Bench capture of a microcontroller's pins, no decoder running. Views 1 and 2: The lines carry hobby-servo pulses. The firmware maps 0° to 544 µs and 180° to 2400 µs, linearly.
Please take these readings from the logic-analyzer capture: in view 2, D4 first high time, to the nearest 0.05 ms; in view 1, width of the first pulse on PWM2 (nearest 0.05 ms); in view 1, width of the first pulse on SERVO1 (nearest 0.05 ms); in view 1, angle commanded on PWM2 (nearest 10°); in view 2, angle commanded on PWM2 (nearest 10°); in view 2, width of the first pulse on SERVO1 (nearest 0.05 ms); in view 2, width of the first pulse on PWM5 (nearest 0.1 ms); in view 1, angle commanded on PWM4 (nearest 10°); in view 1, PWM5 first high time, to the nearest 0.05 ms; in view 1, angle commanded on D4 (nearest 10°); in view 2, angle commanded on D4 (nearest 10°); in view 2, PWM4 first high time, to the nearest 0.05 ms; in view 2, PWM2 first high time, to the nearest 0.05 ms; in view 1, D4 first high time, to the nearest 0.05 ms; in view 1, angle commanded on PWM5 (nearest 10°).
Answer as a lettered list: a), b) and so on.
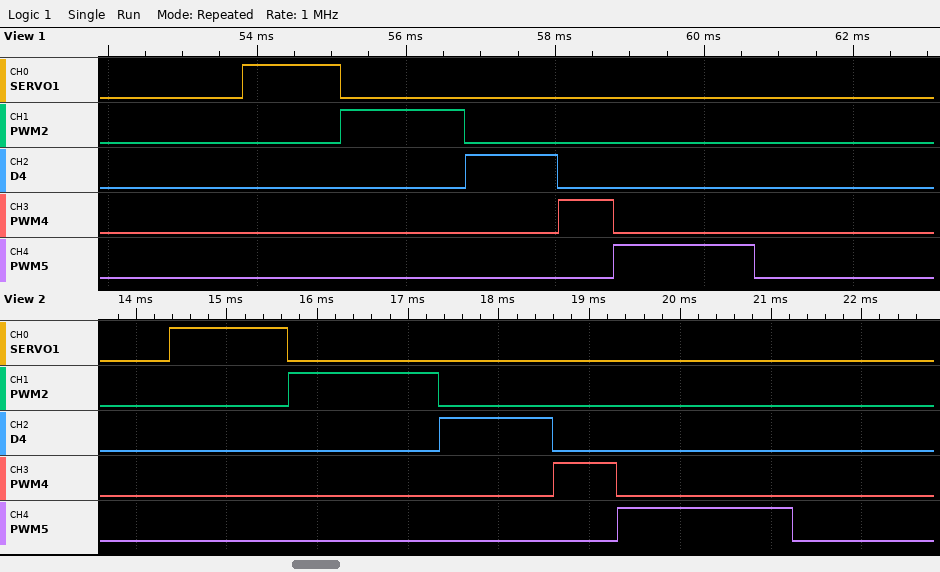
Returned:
a) 1.25 ms
b) 1.65 ms
c) 1.30 ms
d) 110°
e) 110°
f) 1.30 ms
g) 1.9 ms
h) 20°
i) 1.90 ms
j) 70°
k) 70°
l) 0.70 ms
m) 1.65 ms
n) 1.25 ms
o) 130°
